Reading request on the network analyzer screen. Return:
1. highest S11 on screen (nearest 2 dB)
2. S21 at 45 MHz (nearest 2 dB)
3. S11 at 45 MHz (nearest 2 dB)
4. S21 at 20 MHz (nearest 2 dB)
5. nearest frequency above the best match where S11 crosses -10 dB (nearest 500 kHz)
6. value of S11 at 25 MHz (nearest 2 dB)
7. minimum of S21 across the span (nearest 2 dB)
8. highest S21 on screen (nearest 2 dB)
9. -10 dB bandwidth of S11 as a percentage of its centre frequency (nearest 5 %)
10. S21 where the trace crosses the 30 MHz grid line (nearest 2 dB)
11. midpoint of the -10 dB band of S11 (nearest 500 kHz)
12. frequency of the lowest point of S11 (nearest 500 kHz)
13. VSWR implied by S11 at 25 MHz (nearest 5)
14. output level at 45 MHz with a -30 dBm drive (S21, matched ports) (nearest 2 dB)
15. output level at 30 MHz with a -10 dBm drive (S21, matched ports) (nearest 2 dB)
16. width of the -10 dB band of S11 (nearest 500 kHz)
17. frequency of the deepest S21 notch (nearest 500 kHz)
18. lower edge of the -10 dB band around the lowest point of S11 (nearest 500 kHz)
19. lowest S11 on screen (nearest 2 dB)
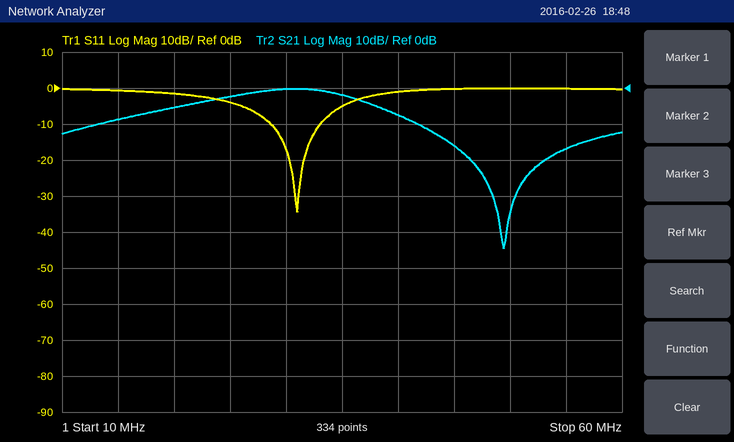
0 dB
-16 dB
0 dB
-6 dB
33.0 MHz
-4 dB
-44 dB
0 dB
15 %
0 dB
31.0 MHz
31.0 MHz
5
-46 dBm
-10 dBm
4.5 MHz
49.5 MHz
28.5 MHz
-34 dB
